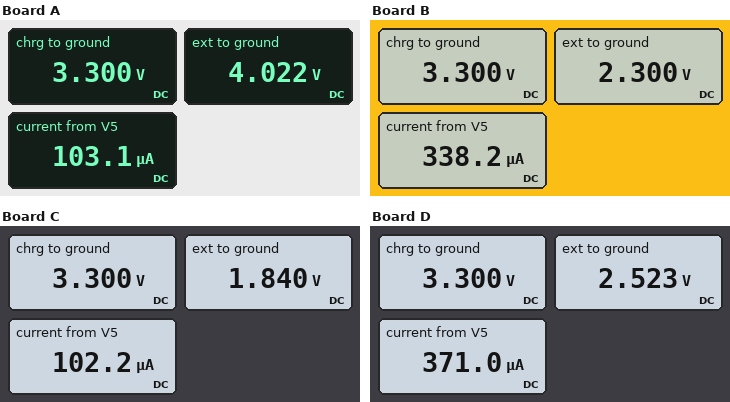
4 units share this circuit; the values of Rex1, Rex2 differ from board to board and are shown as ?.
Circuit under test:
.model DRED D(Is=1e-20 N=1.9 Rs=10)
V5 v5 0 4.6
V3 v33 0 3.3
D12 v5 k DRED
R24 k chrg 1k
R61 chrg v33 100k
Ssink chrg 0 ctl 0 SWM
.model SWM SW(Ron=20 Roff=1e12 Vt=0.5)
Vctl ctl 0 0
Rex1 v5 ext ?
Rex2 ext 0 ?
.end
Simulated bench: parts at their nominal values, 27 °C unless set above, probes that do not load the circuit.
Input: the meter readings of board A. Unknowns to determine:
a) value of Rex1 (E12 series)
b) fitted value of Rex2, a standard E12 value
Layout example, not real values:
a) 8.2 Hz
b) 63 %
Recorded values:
a) 5.6 kΩ
b) 39 kΩ
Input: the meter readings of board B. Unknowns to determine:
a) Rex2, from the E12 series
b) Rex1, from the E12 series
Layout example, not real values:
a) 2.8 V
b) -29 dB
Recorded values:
a) 6.8 kΩ
b) 6.8 kΩ
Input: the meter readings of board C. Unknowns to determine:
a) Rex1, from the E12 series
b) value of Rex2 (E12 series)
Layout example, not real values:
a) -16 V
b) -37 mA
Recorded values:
a) 27 kΩ
b) 18 kΩ
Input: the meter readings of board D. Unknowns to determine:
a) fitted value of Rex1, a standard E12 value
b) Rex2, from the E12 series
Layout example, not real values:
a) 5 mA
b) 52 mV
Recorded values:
a) 5.6 kΩ
b) 6.8 kΩ
